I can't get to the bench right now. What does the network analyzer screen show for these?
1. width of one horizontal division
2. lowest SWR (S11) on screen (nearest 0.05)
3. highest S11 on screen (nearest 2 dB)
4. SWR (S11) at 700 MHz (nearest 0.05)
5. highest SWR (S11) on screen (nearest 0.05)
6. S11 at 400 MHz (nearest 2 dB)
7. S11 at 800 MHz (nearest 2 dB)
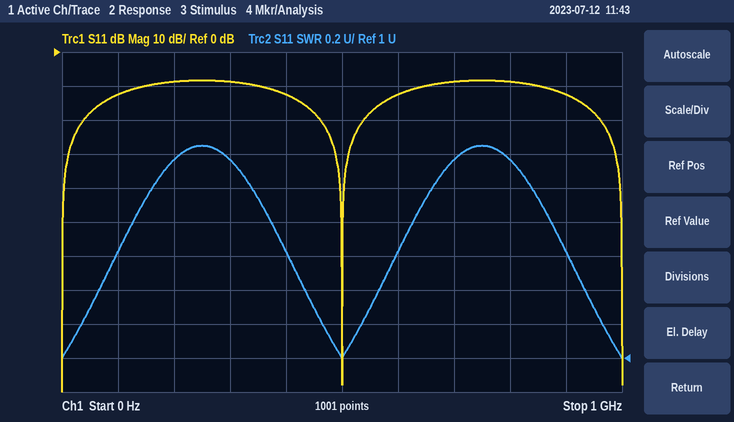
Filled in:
100 MHz
1.00
-8 dB
2.15
2.25
-12 dB
-8 dB
